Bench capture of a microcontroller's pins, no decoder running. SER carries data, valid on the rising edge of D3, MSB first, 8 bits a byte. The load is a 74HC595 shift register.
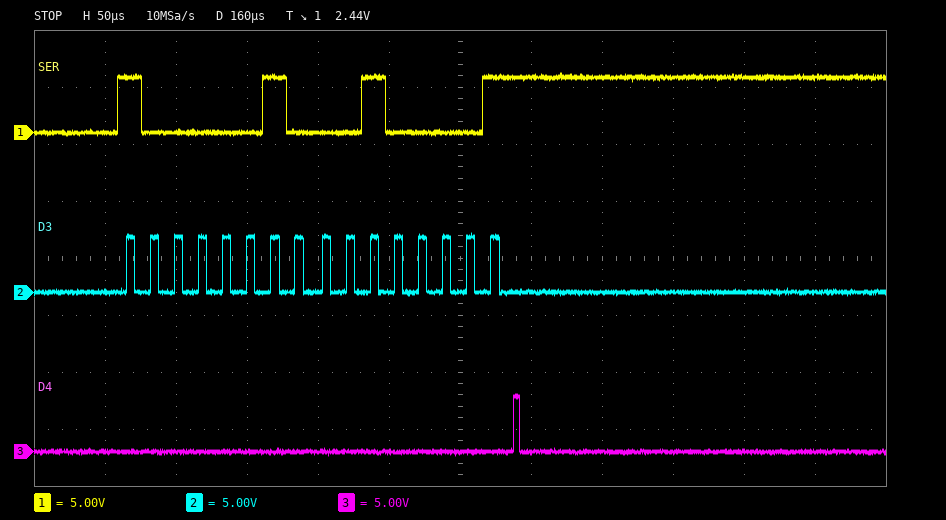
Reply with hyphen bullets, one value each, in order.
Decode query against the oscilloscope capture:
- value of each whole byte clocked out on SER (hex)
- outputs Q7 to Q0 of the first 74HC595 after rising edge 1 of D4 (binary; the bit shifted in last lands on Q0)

- 0x82 0x21
- 00100001
